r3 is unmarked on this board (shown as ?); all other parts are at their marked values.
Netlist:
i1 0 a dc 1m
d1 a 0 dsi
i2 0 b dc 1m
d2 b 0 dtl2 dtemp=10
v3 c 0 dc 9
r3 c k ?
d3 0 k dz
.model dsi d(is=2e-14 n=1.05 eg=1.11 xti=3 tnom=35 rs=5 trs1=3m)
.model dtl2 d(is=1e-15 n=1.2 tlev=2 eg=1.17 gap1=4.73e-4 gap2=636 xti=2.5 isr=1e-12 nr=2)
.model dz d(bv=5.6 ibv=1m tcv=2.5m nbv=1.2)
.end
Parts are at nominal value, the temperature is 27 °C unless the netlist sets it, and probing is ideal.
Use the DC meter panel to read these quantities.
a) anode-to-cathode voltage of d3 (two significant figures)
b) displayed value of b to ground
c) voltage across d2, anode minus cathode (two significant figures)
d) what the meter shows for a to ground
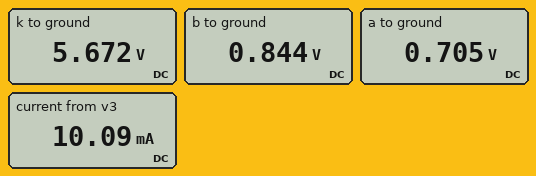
-5.7 V
0.844 V
840 mV
0.705 V
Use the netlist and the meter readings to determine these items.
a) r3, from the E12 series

330 Ω
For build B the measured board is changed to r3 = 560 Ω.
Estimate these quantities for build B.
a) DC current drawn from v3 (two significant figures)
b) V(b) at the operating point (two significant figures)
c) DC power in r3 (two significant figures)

6.0 mA
840 mV
20 mW
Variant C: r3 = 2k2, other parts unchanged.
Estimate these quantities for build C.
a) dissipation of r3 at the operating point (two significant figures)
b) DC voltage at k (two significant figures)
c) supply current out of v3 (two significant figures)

5.2 mW
5.6 V
1.5 mA
